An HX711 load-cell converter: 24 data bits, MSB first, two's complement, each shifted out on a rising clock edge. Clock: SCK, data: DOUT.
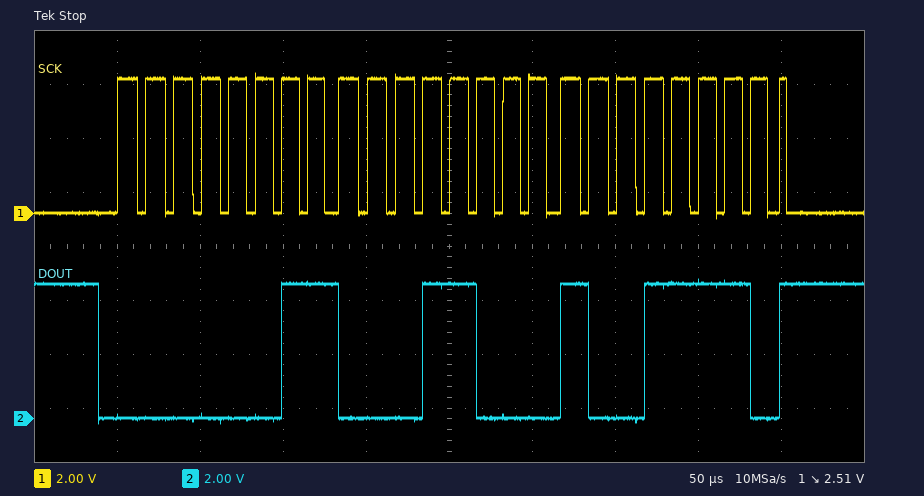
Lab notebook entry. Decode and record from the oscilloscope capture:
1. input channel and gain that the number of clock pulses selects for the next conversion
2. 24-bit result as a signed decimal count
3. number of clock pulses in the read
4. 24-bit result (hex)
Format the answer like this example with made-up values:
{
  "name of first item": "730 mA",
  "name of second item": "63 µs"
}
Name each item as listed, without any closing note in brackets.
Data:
{
  "input channel and gain that the number of clock pulses selects for the next conversion": "channel A, gain 128",
  "24-bit result as a signed decimal count": "202910",
  "number of clock pulses in the read": "25",
  "24-bit result": "0x03189E"
}
